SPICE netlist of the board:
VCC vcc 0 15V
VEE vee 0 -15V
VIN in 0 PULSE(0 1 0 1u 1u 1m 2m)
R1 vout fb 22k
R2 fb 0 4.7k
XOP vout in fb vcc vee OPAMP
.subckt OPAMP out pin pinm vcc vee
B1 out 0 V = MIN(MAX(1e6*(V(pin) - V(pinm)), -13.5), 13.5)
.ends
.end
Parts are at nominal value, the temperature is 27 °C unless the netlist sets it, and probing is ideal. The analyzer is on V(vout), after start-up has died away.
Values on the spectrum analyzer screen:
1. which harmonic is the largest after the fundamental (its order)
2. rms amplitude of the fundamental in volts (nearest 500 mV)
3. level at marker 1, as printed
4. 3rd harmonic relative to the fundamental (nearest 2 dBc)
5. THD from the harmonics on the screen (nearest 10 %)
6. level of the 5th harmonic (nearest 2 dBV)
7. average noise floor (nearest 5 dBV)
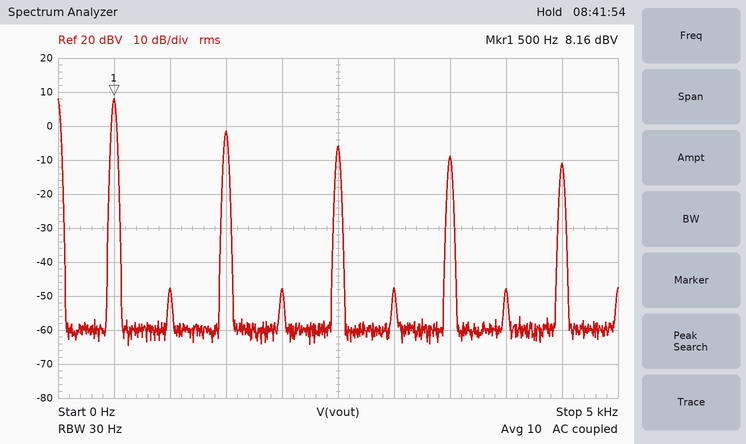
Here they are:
3
2.5 V
8.16 dBV
-10 dBc
40 %
-6 dBV
-60 dBV
